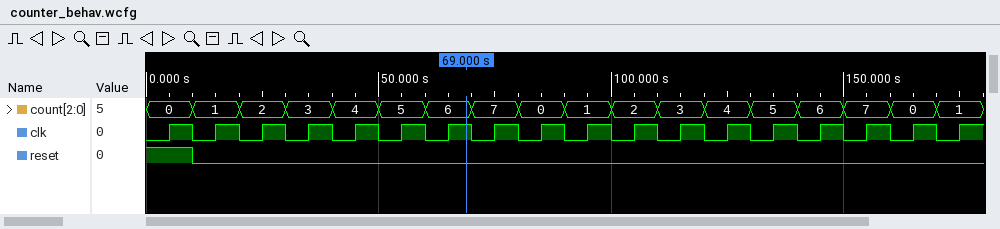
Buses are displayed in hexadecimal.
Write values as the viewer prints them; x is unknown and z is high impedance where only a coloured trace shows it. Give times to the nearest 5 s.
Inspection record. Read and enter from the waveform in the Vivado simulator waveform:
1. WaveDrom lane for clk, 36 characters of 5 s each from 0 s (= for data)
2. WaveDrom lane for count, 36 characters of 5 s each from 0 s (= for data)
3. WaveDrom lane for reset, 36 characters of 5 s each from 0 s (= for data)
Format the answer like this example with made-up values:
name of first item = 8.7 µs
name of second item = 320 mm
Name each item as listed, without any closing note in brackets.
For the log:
WaveDrom lane for clk, 36 characters of 5 s each from 0 s = {name: 'clk', wave: '010101010101010101010101010101010101'}
WaveDrom lane for count, 36 characters of 5 s each from 0 s = {name: 'count', wave: '=.=.=.=.=.=.=.=.=.=.=.=.=.=.=.=.=.=.', data: '0 1 2 3 4 5 6 7 0 1 2 3 4 5 6 7 0 1'}
WaveDrom lane for reset, 36 characters of 5 s each from 0 s = {name: 'reset', wave: '1.0.................................'}
